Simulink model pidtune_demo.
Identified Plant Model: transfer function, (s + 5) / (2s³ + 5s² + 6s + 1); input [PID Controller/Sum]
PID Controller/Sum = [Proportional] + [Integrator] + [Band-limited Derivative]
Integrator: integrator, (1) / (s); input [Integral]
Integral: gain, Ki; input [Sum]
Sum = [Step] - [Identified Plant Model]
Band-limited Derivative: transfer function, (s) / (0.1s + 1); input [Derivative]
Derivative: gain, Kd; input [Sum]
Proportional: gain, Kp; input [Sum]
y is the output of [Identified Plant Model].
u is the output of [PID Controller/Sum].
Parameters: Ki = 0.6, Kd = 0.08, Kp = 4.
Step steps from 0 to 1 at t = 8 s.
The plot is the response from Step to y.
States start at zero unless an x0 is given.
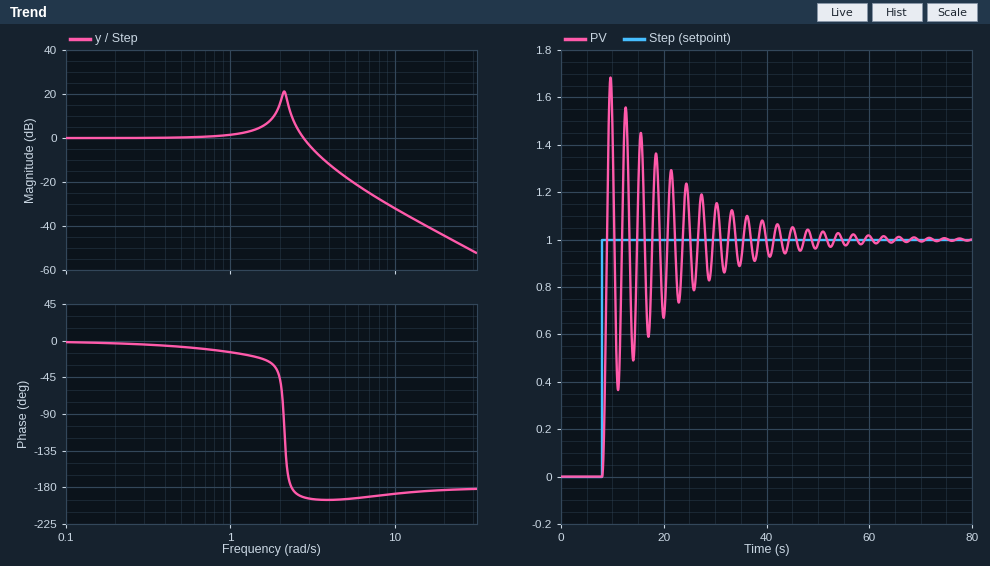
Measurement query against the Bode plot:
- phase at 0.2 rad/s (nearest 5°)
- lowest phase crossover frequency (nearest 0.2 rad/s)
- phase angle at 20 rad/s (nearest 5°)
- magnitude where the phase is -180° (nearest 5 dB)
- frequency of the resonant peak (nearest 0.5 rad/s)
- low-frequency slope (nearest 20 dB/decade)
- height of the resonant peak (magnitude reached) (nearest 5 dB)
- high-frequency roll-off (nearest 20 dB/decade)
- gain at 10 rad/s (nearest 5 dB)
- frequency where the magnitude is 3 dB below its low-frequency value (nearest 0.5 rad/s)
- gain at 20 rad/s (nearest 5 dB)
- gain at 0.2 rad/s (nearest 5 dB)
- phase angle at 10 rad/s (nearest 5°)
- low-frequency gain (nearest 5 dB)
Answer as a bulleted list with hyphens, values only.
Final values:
- -5°
- 2.4 rad/s
- -185°
- 10 dB
- 2.0 rad/s
- 0 dB/decade
- 20 dB
- -40 dB/decade
- -30 dB
- 3.0 rad/s
- -45 dB
- 0 dB
- -190°
- 0 dB
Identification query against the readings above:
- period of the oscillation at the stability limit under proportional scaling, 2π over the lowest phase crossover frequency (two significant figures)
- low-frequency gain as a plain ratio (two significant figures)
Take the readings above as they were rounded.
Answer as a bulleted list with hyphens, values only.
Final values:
- 2.6 s
- 1.0
